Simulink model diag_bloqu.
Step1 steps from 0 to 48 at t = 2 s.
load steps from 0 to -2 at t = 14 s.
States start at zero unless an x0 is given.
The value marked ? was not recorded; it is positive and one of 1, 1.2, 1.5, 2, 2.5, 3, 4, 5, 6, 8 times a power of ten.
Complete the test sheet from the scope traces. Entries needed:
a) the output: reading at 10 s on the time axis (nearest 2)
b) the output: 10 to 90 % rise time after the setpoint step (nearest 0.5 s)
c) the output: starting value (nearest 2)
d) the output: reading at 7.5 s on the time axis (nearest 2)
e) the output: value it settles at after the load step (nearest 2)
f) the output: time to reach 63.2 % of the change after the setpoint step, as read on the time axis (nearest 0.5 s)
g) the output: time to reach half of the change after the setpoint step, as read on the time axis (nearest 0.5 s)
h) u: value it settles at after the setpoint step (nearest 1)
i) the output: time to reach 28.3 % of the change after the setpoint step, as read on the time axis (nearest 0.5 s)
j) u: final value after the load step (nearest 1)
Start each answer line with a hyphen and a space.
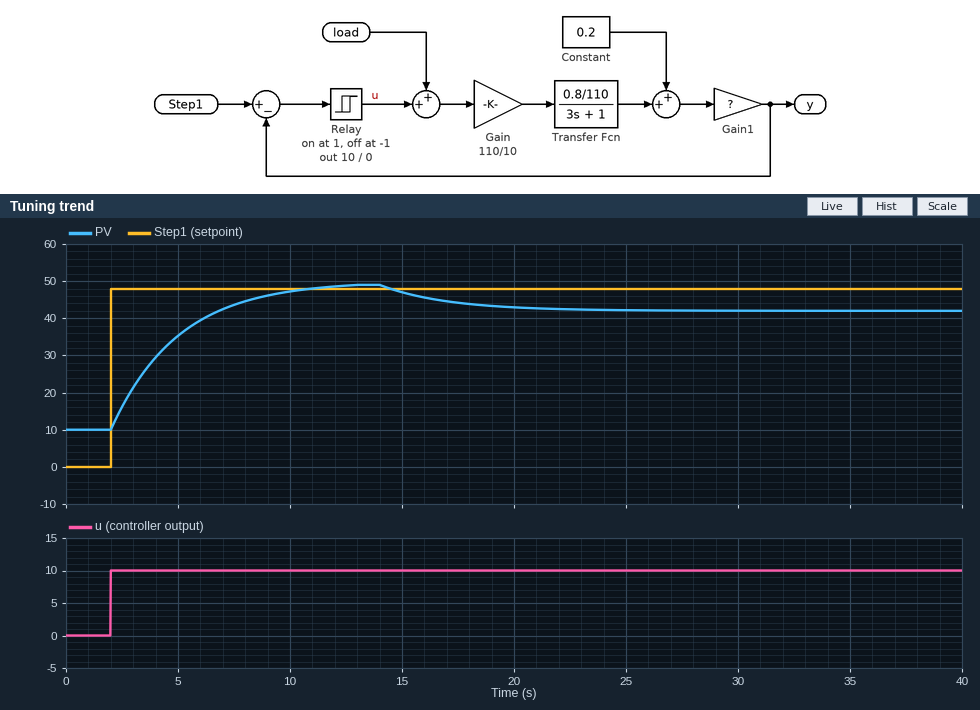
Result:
- 48
- 6.0 s
- 10
- 44
- 42
- 5.0 s
- 4.0 s
- 10
- 3.0 s
- 10
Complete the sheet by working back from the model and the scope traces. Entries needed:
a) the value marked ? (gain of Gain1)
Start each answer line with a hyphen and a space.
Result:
- 50
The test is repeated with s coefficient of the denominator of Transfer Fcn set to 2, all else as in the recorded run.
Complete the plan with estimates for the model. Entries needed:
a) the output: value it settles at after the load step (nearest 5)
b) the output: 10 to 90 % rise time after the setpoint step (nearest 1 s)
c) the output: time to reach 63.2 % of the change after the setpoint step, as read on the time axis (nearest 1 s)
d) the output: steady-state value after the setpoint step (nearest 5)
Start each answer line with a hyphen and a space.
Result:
- 40
- 4 s
- 4 s
- 50
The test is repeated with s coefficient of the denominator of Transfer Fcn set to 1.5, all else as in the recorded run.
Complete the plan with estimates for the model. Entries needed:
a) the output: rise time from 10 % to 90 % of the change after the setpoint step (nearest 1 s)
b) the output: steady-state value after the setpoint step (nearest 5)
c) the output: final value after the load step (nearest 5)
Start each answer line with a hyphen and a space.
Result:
- 3 s
- 50
- 40
